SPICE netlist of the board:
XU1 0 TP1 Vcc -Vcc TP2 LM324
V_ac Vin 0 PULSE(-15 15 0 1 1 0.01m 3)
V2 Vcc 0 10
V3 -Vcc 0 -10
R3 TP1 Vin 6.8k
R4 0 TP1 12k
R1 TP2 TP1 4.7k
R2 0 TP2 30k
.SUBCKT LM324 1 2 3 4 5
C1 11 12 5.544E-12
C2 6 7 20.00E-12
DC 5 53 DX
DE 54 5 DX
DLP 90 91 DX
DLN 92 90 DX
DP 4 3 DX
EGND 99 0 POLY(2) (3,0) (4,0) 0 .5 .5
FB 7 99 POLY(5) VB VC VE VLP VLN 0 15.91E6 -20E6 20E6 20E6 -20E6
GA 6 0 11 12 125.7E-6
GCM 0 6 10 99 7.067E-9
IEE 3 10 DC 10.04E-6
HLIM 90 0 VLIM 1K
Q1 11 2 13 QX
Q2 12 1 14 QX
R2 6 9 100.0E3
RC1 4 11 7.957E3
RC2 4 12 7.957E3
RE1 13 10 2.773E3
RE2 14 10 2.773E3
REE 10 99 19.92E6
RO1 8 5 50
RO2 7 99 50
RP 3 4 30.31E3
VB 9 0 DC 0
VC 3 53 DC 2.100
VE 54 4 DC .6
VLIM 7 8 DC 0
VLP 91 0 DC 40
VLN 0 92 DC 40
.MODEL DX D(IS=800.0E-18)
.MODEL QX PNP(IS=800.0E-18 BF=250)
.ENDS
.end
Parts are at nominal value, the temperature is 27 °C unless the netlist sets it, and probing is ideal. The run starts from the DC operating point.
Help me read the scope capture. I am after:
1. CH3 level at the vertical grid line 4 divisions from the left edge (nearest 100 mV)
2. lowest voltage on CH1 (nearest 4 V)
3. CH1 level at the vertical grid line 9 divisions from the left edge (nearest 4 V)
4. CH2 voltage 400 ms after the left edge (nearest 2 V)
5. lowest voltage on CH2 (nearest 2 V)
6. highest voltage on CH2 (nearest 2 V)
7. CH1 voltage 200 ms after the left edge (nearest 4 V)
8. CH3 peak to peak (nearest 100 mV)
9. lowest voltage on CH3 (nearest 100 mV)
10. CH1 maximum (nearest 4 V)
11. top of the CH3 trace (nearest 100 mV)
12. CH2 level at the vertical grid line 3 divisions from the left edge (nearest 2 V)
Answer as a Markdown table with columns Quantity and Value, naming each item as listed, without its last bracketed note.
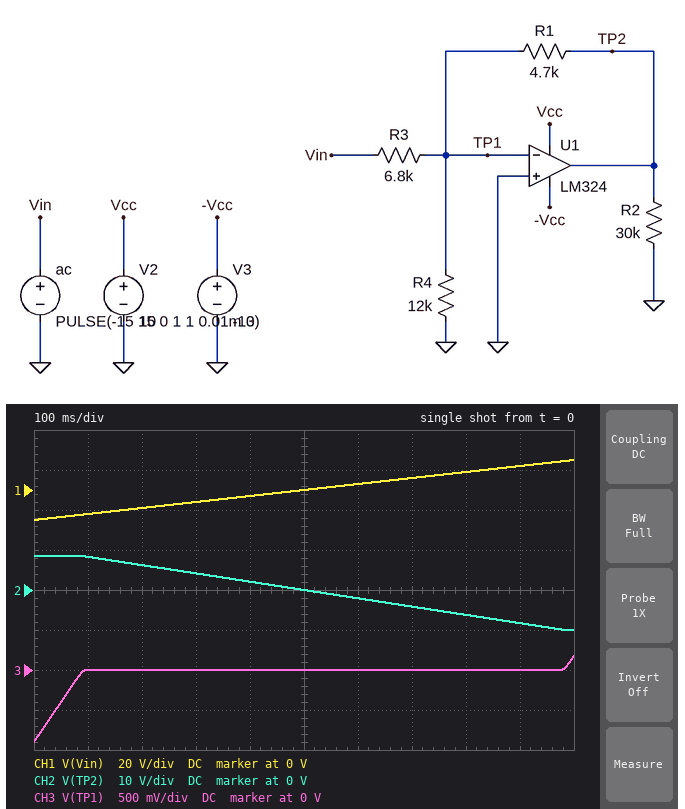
| Quantity | Value |
|---|---|
| CH3 level at the vertical grid line 4 divisions from the left edge | 0 V |
| lowest voltage on CH1 | -16 V |
| CH1 level at the vertical grid line 9 divisions from the left edge | 12 V |
| CH2 voltage 400 ms after the left edge | 2 V |
| lowest voltage on CH2 | -10 V |
| highest voltage on CH2 | 8 V |
| CH1 voltage 200 ms after the left edge | -8 V |
| CH3 peak to peak | 1.1 V |
| lowest voltage on CH3 | -900 mV |
| CH1 maximum | 16 V |
| top of the CH3 trace | 200 mV |
| CH2 level at the vertical grid line 3 divisions from the left edge | 4 V |
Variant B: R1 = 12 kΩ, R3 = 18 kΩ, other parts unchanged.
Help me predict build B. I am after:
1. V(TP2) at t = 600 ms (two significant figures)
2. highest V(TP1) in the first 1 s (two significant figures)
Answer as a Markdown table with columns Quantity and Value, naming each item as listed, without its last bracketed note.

| Quantity | Value |
|---|---|
| V(TP2) at t = 600 ms | -2.0 V |
| highest V(TP1) in the first 1 s | 17 mV |
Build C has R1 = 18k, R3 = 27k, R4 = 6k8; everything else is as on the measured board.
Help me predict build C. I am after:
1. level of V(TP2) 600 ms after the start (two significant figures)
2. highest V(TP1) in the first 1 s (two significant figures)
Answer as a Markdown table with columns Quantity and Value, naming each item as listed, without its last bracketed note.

| Quantity | Value |
|---|---|
| level of V(TP2) 600 ms after the start | -2.0 V |
| highest V(TP1) in the first 1 s | 12 mV |
